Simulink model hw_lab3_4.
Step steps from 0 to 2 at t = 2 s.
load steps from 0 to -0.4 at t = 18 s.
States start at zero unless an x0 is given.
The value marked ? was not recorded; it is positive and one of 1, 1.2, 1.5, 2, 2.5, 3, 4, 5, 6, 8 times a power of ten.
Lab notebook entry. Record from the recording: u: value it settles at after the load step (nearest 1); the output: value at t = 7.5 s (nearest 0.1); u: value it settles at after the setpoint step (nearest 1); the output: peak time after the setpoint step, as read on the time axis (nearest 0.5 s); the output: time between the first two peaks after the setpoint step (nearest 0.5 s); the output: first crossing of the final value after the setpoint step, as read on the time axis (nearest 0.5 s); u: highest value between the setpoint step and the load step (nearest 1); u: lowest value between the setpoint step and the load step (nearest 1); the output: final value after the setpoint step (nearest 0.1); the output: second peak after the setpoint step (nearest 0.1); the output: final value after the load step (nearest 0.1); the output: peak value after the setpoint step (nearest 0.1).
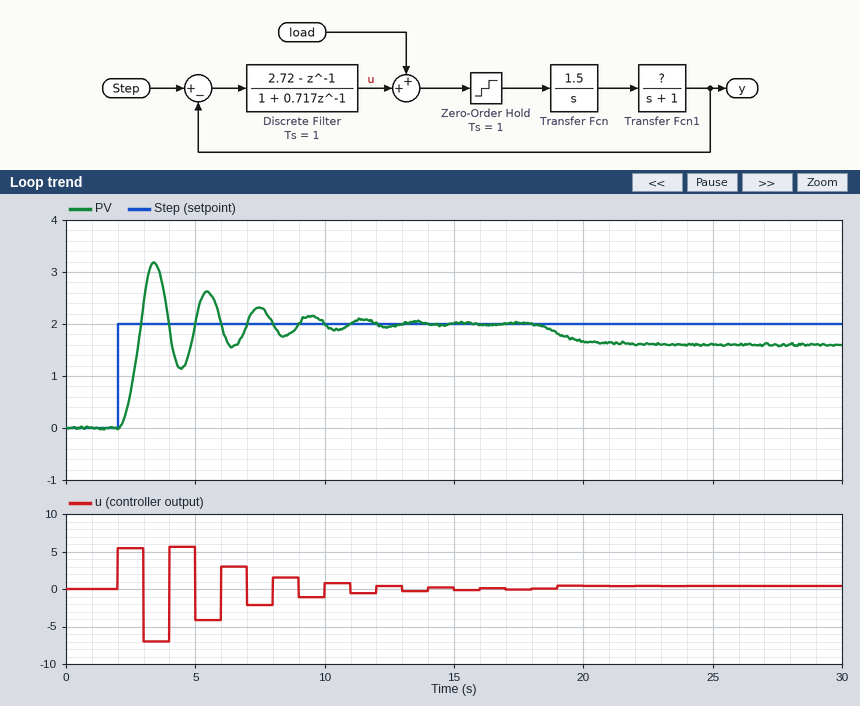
0
2.3
0
3.5 s
2.0 s
3.0 s
6
-7
2.0
2.6
1.6
3.2
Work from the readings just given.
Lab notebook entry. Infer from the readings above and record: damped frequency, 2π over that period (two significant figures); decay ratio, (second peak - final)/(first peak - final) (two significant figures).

3.1 rad/s
0.50
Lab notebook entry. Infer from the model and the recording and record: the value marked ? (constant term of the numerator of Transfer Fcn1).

0.8
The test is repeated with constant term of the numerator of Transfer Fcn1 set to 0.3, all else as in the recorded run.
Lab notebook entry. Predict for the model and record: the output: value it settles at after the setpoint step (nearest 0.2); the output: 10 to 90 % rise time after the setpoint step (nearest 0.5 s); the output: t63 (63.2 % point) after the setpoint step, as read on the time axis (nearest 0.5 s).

2.0
3.0 s
3.5 s
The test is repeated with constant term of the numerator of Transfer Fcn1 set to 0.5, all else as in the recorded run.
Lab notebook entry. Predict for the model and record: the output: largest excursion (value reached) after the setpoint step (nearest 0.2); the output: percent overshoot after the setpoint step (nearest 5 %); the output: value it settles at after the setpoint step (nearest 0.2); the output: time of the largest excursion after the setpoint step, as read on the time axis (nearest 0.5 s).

2.2
10 %
2.0
5.5 s
